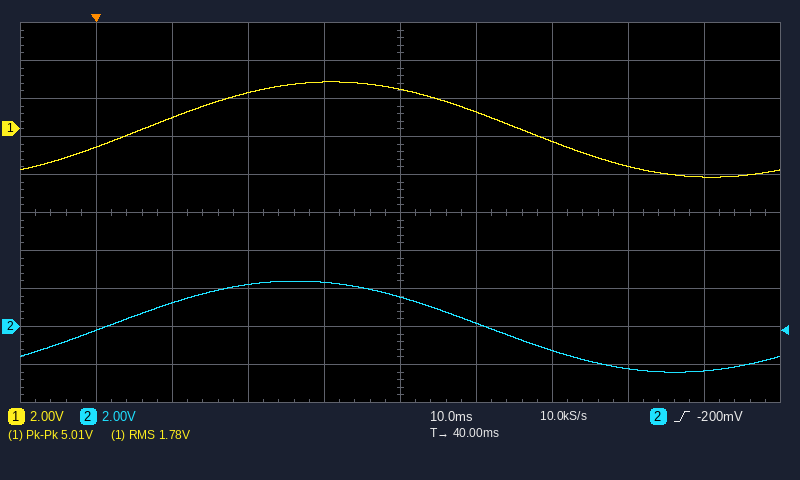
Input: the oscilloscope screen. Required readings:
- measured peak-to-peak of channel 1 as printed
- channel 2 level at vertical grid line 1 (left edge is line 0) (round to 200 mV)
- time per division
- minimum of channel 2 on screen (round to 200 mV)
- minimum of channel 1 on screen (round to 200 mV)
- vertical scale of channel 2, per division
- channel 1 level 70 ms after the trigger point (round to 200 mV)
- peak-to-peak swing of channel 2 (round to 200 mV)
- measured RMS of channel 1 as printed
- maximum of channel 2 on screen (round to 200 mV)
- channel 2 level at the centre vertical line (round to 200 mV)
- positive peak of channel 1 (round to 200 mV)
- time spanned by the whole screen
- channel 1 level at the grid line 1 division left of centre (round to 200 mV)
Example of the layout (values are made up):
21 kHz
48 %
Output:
5.01 V
-200 mV
10 ms
-2.4 V
-2.6 V
2 V
-2.0 V
4.8 V
1.78 V
2.4 V
1.6 V
2.4 V
100 ms
2.4 V
